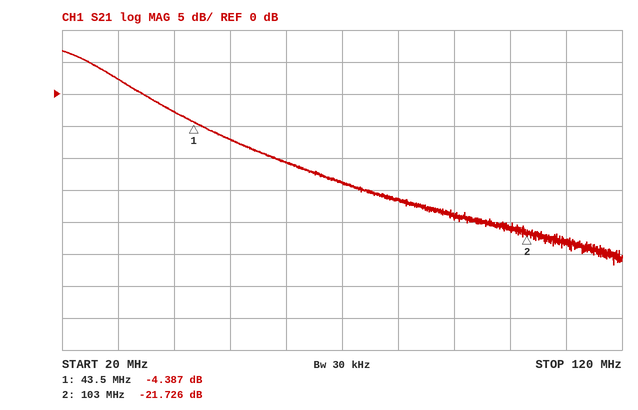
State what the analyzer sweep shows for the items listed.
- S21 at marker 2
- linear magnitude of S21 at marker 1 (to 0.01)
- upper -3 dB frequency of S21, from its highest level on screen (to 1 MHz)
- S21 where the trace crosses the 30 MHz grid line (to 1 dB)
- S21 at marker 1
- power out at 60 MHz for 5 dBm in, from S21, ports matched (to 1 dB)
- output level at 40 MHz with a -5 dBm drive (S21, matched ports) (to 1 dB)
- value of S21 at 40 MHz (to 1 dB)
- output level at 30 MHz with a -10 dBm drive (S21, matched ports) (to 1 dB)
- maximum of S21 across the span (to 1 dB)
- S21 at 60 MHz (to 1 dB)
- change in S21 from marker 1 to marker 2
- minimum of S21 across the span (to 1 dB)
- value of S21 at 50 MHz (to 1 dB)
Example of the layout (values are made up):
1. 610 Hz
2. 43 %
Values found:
1. -21.726 dB
2. 0.60
3. 27 MHz
4. 2 dB
5. -4.387 dB
6. -6 dBm
7. -8 dBm
8. -3 dB
9. -8 dBm
10. 7 dB
11. -11 dB
12. -17.339 dB
13. -27 dB
14. -7 dB
